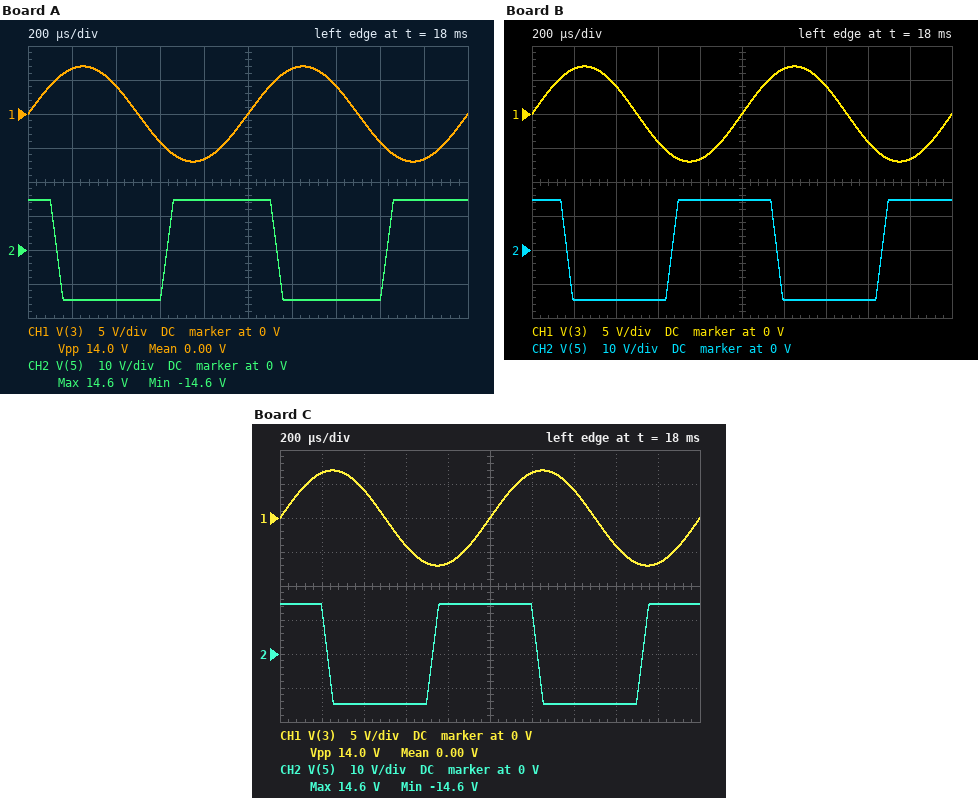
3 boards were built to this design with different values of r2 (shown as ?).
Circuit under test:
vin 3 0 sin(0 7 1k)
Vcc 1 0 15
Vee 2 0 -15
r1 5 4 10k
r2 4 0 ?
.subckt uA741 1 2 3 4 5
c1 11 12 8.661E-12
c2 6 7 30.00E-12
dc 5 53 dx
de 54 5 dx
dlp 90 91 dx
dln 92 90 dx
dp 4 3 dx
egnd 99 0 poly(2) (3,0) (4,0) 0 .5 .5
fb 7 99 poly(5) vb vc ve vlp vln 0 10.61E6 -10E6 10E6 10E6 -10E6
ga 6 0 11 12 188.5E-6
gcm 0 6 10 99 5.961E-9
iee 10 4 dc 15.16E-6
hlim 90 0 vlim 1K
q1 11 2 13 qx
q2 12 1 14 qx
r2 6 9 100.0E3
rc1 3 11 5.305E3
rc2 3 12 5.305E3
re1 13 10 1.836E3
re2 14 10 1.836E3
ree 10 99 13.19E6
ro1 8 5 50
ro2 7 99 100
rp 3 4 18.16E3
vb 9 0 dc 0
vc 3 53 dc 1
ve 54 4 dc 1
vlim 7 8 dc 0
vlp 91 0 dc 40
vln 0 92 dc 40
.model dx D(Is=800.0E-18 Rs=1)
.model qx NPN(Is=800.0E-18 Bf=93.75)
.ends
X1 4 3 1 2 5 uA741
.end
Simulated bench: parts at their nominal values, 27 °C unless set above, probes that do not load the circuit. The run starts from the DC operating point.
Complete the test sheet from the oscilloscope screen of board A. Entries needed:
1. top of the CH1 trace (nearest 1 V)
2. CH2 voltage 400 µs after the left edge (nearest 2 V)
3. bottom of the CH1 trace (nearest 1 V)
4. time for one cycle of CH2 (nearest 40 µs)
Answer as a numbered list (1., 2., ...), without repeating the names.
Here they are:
1. 7 V
2. -14 V
3. -7 V
4. 1.00 ms
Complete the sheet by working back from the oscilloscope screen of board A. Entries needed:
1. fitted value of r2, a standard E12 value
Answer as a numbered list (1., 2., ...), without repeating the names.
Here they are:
1. 3.9 kΩ
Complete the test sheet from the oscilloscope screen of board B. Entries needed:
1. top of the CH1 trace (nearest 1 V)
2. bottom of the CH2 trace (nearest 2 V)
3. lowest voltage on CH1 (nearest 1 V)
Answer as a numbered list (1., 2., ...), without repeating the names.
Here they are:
1. 7 V
2. -14 V
3. -7 V
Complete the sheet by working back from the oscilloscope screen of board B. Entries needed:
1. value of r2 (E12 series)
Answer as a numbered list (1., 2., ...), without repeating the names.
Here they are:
1. 5.6 kΩ
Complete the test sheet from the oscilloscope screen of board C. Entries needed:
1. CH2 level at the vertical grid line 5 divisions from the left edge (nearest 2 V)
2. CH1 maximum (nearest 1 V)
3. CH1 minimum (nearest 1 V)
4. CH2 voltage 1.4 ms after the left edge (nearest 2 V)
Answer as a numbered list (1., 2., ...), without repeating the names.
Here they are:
1. 14 V
2. 7 V
3. -7 V
4. -14 V
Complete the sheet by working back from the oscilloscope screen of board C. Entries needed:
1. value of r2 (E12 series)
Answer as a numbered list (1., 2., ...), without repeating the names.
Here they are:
1. 8.2 kΩ
